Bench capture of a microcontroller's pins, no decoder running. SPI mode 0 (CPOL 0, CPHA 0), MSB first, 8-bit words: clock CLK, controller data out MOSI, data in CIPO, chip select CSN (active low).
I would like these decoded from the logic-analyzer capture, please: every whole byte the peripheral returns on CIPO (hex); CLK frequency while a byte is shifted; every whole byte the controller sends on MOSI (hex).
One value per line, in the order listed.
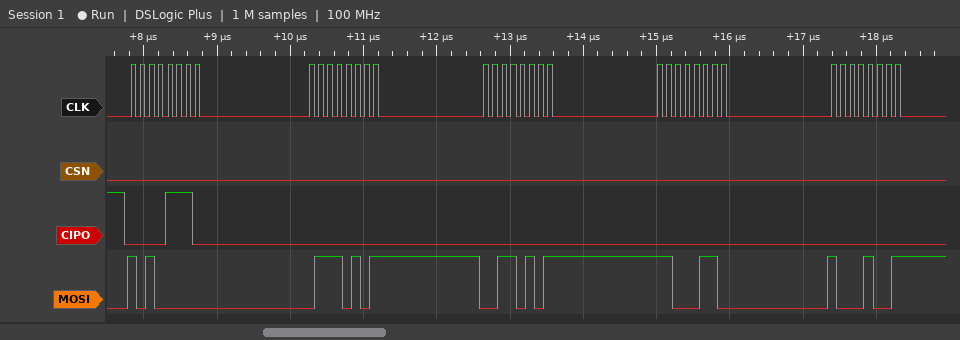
0E 00 00 00 00
8 MHz
A0 75 35 C6 89
